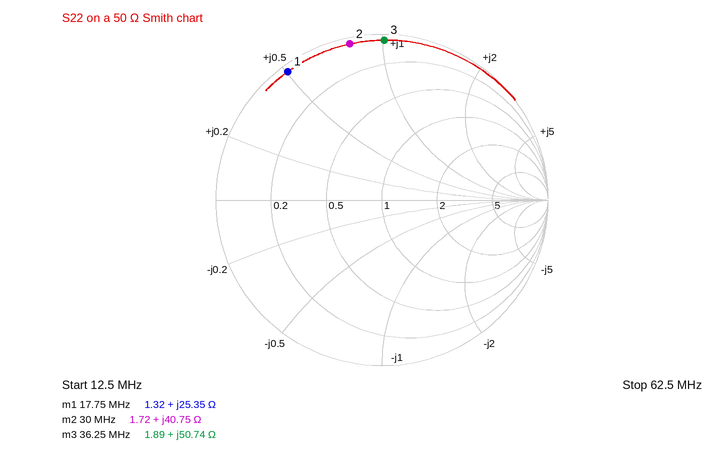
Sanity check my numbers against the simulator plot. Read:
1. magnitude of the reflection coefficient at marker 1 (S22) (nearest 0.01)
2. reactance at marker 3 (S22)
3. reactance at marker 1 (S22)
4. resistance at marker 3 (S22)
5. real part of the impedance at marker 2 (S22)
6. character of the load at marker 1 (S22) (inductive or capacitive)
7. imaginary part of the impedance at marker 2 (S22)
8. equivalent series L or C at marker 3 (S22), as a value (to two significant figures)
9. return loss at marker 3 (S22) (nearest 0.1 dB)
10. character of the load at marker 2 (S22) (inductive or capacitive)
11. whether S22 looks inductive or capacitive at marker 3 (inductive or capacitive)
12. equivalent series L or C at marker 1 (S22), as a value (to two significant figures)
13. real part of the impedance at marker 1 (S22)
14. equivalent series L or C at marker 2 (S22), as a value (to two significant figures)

0.96
+50.74 Ω
+25.35 Ω
1.89 Ω
1.72 Ω
inductive
+40.75 Ω
220 nH
0.3 dB
inductive
inductive
230 nH
1.32 Ω
220 nH
